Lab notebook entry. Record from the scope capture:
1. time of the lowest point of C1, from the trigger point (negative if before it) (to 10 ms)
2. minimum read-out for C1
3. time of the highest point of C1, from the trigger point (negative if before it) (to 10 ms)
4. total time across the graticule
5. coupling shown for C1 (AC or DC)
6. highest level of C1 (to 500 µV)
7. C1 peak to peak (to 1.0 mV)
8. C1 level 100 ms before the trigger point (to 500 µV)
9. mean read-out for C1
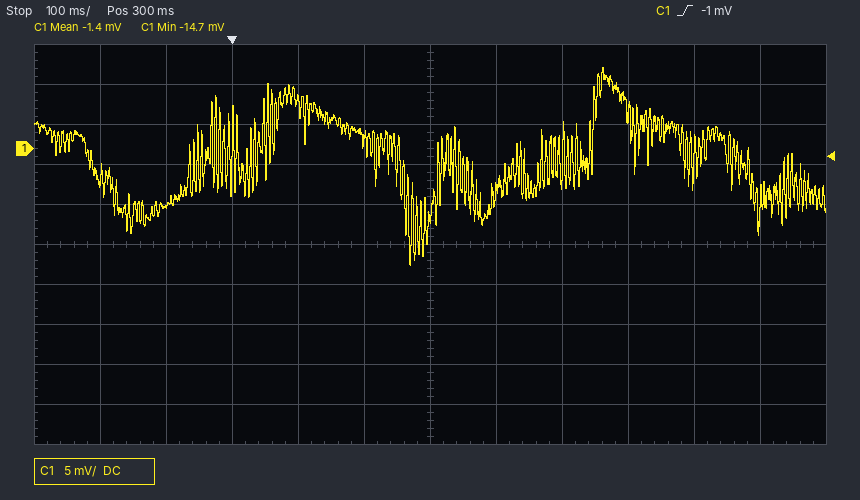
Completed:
+270 ms
-14.7 mV
+560 ms
1.2 s
DC
10.0 mV
25.0 mV
-7.0 mV
-1.4 mV
